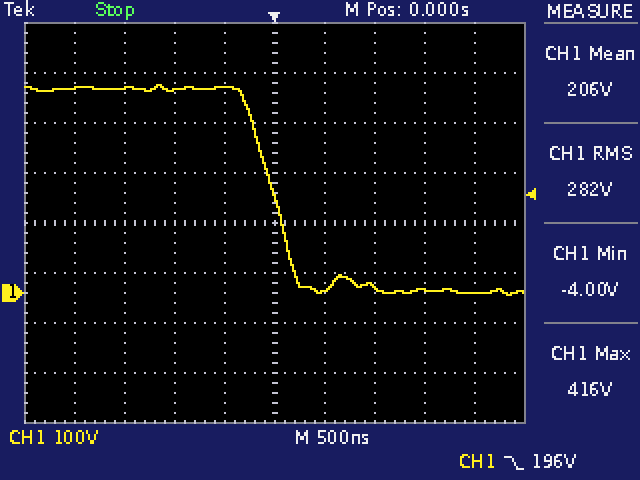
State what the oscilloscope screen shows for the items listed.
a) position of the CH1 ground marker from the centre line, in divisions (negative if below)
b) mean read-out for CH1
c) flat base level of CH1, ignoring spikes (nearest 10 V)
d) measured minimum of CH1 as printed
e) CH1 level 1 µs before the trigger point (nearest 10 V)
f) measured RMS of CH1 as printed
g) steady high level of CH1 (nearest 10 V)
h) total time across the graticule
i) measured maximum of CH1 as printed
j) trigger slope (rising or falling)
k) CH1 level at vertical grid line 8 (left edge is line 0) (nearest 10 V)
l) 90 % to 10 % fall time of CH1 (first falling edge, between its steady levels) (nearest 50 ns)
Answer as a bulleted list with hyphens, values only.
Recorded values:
- -1.4 div
- 206 V
- 0 V
- -4.00 V
- 410 V
- 282 V
- 410 V
- 5 µs
- 416 V
- falling
- 10 V
- 450 ns
